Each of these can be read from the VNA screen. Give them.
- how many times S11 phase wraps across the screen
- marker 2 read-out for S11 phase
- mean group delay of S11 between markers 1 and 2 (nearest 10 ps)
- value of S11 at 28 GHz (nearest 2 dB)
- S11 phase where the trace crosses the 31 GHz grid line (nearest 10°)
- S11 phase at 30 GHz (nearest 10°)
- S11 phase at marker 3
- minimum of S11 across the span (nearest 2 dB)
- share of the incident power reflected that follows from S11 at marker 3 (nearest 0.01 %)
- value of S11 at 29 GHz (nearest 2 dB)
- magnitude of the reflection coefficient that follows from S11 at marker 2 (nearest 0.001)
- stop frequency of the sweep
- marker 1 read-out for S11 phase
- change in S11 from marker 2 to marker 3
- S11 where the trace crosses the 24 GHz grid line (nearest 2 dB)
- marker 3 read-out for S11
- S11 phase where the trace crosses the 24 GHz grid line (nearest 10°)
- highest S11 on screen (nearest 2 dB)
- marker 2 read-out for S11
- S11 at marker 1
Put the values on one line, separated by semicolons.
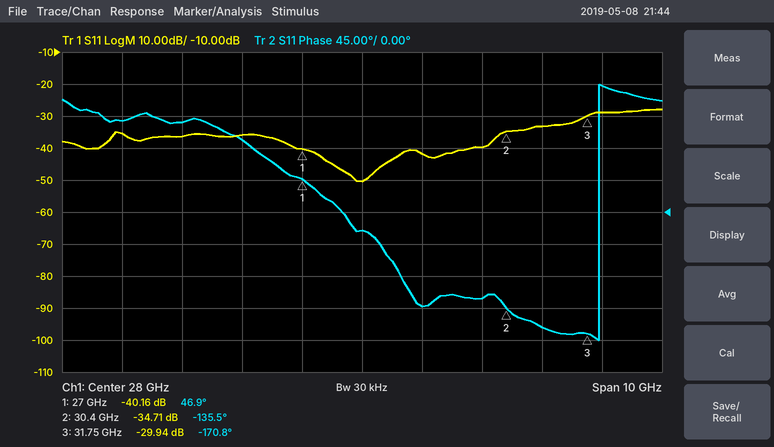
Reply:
1; -135.5°; 150 ps; -50 dB; -160°; -120°; -170.8°; -50 dB; 0.10 %; -42 dB; 0.018; 33 GHz; 46.9°; 4.77 dB; -36 dB; -29.94 dB; 130°; -28 dB; -34.71 dB; -40.16 dB
